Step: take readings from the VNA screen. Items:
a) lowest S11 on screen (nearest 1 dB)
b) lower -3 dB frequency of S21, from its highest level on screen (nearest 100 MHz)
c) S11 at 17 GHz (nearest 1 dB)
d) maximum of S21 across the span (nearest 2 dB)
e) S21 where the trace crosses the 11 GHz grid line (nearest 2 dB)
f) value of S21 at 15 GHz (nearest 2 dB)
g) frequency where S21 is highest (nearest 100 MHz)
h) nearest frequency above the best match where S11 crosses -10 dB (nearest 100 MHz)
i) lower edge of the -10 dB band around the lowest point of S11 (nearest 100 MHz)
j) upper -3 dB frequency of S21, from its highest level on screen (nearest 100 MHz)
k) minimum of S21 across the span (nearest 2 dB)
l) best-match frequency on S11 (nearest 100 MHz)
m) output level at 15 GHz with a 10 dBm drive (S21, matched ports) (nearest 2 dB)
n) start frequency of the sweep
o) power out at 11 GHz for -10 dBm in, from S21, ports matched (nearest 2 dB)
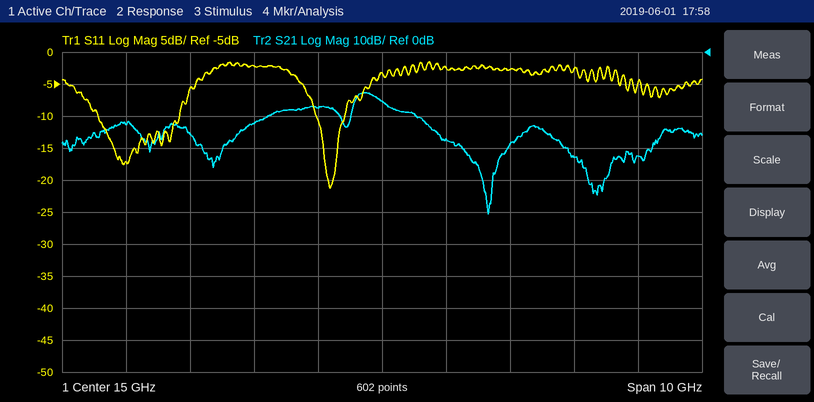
-21 dB
14.6 GHz
-3 dB
-12 dB
-22 dB
-16 dB
14.7 GHz
14.4 GHz
14.0 GHz
15.0 GHz
-50 dB
14.2 GHz
-6 dBm
10 GHz
-32 dBm
